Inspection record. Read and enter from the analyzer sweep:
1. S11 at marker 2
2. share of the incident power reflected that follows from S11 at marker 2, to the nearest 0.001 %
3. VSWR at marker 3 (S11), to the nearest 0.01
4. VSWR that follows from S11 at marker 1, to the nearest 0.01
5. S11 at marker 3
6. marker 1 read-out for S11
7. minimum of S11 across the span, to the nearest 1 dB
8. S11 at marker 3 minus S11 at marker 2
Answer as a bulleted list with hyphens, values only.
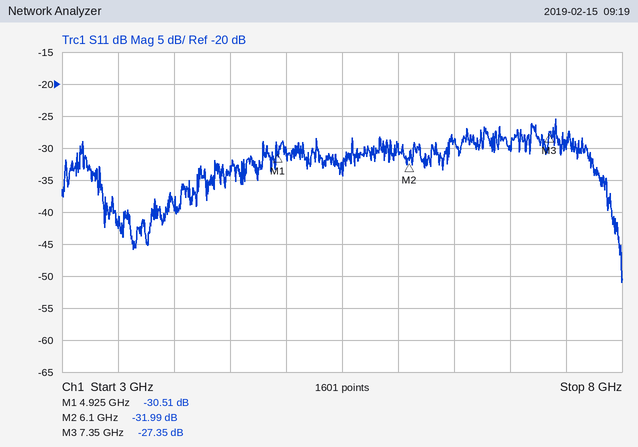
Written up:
- -31.99 dB
- 0.063 %
- 1.09
- 1.06
- -27.35 dB
- -30.51 dB
- -51 dB
- 4.64 dB
